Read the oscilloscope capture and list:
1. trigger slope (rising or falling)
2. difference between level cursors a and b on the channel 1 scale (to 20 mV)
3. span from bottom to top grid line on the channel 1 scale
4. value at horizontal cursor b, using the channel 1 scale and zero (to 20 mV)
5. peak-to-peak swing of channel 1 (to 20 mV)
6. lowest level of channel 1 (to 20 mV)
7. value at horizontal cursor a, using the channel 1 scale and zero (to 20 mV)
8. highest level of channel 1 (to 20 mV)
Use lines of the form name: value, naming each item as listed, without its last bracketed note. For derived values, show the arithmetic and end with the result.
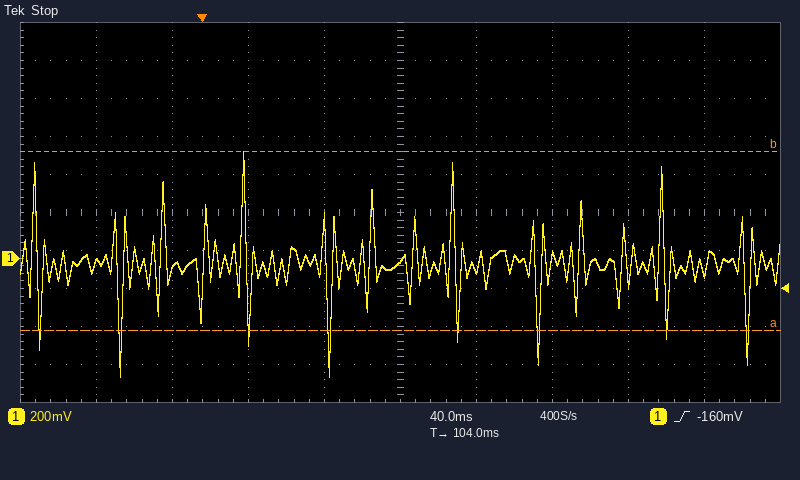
trigger slope: rising
difference between level cursors a and b on the channel 1 scale: 940 mV
span from bottom to top grid line on the channel 1 scale: 2 V
value at horizontal cursor b, using the channel 1 scale and zero: 560 mV
peak-to-peak swing of channel 1: 560 mV − (-620 mV) = 1.18 V
lowest level of channel 1: -620 mV
value at horizontal cursor a, using the channel 1 scale and zero: -380 mV
highest level of channel 1: 560 mV
